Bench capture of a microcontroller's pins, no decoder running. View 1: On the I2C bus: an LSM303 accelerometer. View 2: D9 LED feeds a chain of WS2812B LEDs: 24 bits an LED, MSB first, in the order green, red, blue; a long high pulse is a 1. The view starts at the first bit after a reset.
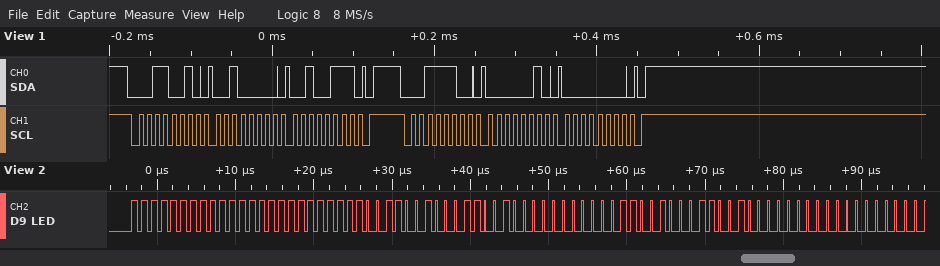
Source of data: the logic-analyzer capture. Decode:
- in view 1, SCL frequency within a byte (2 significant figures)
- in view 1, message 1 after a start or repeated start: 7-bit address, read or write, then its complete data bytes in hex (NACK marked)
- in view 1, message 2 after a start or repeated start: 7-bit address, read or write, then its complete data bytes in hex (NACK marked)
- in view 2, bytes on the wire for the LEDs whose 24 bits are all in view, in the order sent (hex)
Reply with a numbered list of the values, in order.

1. 100 kHz
2. 0x19 write: 20 27
3. 0x1E write: 02 00
4. FF FF FF 32 32 00 32 32 00
